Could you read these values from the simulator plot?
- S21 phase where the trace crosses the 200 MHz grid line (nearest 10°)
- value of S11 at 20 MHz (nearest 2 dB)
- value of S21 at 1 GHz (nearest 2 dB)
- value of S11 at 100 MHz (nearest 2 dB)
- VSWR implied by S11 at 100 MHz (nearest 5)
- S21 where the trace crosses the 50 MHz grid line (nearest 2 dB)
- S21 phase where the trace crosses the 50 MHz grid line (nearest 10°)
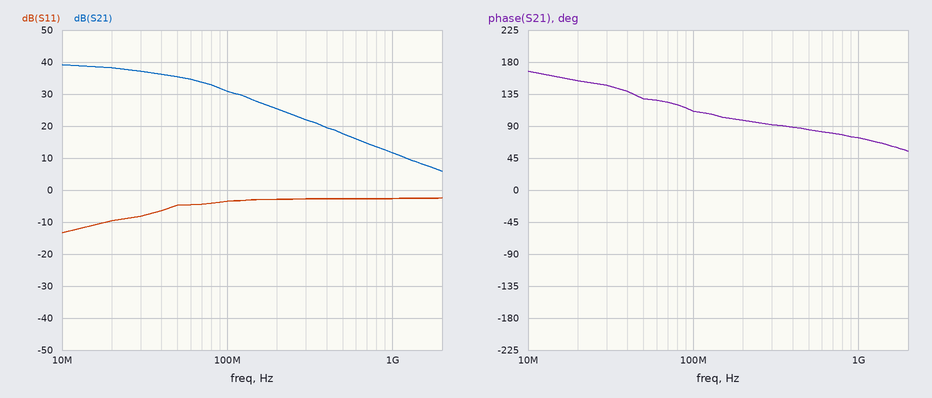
100°
-10 dB
12 dB
-4 dB
5
36 dB
130°
